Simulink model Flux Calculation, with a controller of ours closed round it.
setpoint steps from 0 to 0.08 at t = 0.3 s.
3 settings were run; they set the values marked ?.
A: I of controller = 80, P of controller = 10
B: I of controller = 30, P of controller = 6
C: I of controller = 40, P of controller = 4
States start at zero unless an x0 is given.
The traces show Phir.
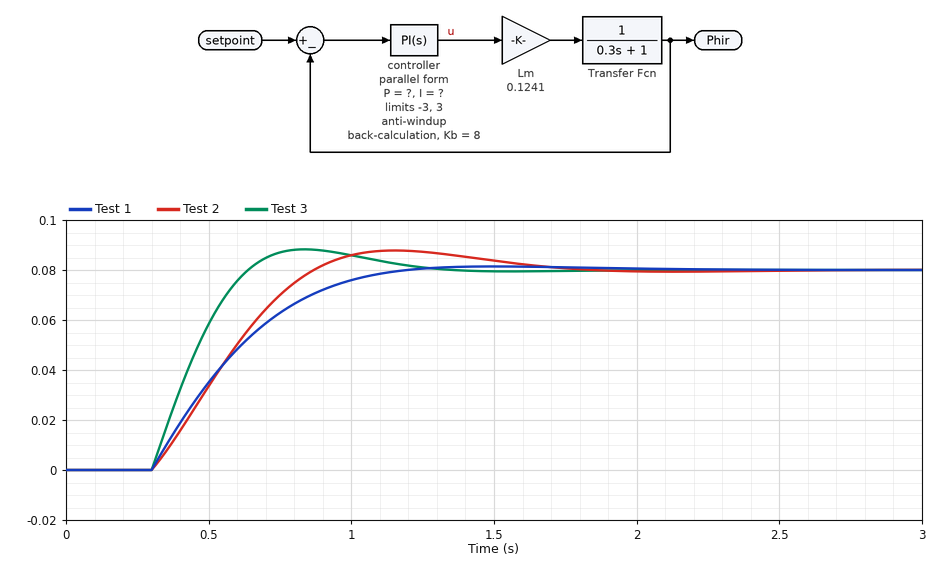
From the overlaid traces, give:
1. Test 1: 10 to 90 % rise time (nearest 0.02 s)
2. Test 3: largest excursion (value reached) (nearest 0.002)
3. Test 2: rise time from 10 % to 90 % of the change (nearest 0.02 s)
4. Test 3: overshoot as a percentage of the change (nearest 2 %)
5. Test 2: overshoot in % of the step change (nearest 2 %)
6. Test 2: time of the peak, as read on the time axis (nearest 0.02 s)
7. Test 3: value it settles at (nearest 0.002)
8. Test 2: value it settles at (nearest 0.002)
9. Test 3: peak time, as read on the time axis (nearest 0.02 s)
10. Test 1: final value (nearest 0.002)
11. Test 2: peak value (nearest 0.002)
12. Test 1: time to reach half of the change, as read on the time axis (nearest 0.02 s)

0.56 s
0.088
0.42 s
10 %
10 %
1.16 s
0.080
0.080
0.84 s
0.080
0.088
0.54 s
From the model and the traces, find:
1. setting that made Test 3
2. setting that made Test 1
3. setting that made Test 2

A
B
C
